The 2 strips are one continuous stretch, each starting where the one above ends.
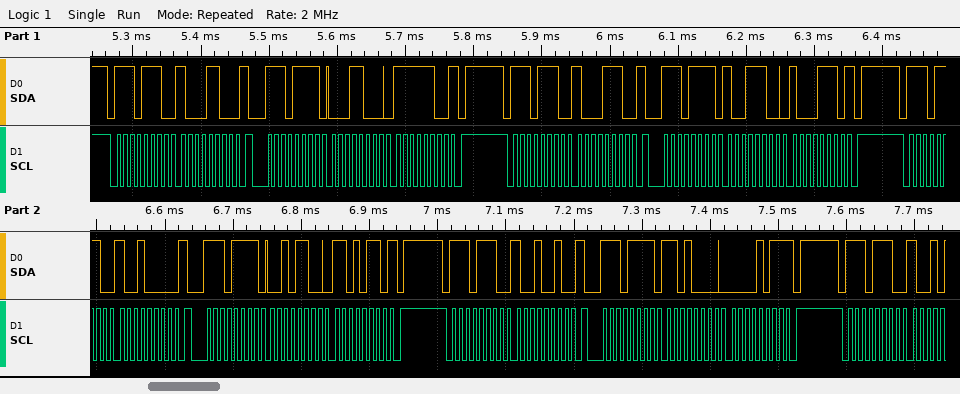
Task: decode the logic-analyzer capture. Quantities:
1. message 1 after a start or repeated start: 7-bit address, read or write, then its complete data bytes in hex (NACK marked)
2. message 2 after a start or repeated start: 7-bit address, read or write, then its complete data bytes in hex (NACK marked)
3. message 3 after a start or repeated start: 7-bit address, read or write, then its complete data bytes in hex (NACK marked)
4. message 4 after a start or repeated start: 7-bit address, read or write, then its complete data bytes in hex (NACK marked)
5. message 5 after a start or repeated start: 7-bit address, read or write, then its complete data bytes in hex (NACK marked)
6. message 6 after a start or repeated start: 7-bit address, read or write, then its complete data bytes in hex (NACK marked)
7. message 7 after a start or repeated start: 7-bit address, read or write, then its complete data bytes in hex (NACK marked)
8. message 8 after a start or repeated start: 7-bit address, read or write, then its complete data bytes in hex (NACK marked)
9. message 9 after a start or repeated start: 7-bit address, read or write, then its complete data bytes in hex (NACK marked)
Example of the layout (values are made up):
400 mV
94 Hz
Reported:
0x77 write: 8C
0x77 read: 18 FC NACK
0x77 write: 8E
0x77 read: 9C 8E NACK
0x77 write: 90
0x77 read: 2C D6 NACK
0x77 write: 92
0x77 read: D0 0B NACK
0x77 write
